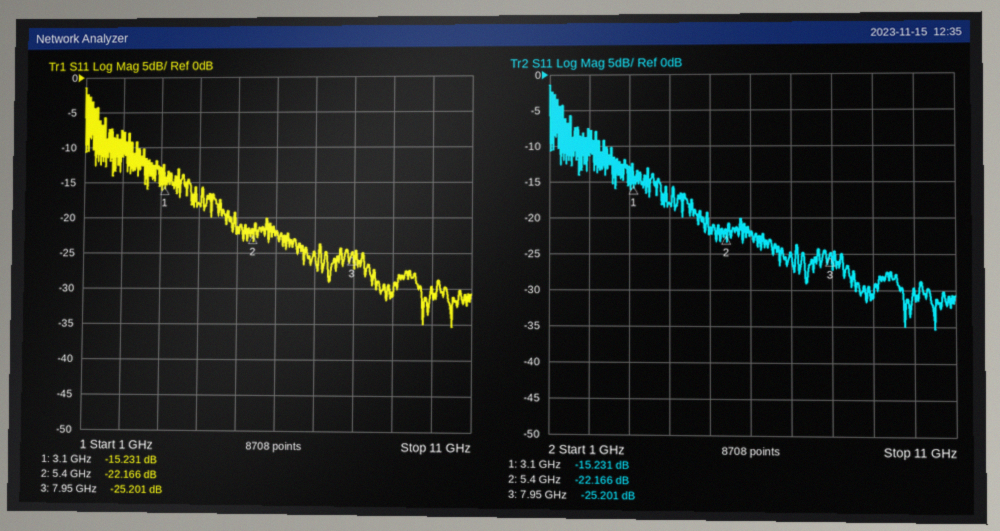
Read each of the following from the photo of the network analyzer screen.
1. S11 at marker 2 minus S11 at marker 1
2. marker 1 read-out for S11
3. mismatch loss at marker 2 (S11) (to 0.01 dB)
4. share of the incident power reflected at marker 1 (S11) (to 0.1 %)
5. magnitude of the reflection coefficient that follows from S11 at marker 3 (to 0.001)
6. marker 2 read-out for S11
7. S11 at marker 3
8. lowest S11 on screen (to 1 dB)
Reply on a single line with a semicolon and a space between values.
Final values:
-6.935 dB; -15.231 dB; 0.03 dB; 3.0 %; 0.055; -22.166 dB; -25.201 dB; -35 dB
